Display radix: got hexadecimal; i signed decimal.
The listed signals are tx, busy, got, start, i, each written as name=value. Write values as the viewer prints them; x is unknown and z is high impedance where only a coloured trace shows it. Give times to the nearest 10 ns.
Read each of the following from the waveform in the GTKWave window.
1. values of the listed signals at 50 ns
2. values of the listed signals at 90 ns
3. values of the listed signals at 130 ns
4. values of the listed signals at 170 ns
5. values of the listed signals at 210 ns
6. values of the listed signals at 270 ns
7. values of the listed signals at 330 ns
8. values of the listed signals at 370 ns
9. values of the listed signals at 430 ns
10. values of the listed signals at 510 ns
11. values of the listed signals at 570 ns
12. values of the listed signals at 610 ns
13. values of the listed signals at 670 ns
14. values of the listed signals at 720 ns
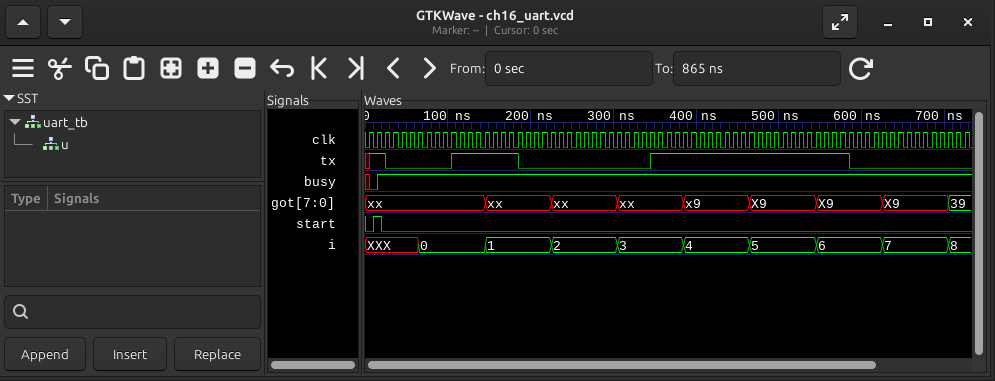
tx=0, busy=1, got=xx, start=0, i=XXX
tx=0, busy=1, got=xx, start=0, i=0
tx=1, busy=1, got=xx, start=0, i=0
tx=1, busy=1, got=xx, start=0, i=1
tx=0, busy=1, got=xx, start=0, i=1
tx=0, busy=1, got=xx, start=0, i=2
tx=0, busy=1, got=xx, start=0, i=3
tx=1, busy=1, got=xx, start=0, i=3
tx=1, busy=1, got=x9, start=0, i=4
tx=1, busy=1, got=X9, start=0, i=5
tx=1, busy=1, got=X9, start=0, i=6
tx=0, busy=1, got=X9, start=0, i=6
tx=0, busy=1, got=X9, start=0, i=7
tx=0, busy=1, got=39, start=0, i=8
